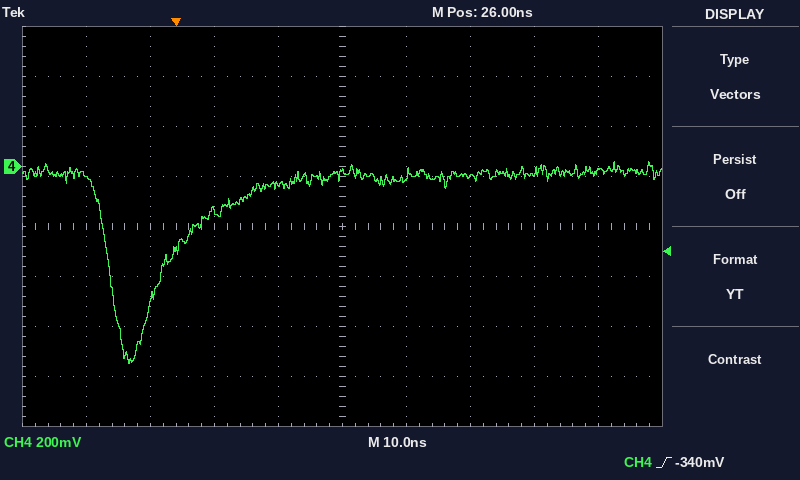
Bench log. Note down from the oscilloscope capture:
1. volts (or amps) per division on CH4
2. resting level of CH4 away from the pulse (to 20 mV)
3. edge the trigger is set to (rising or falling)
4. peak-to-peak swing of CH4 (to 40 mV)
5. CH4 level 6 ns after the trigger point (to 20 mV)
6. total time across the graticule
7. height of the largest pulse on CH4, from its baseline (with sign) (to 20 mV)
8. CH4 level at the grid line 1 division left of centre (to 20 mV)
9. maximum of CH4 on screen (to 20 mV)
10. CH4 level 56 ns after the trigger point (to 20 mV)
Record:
200 mV
-40 mV
rising
800 mV
-180 mV
100 ns
-760 mV
-80 mV
20 mV
-20 mV
